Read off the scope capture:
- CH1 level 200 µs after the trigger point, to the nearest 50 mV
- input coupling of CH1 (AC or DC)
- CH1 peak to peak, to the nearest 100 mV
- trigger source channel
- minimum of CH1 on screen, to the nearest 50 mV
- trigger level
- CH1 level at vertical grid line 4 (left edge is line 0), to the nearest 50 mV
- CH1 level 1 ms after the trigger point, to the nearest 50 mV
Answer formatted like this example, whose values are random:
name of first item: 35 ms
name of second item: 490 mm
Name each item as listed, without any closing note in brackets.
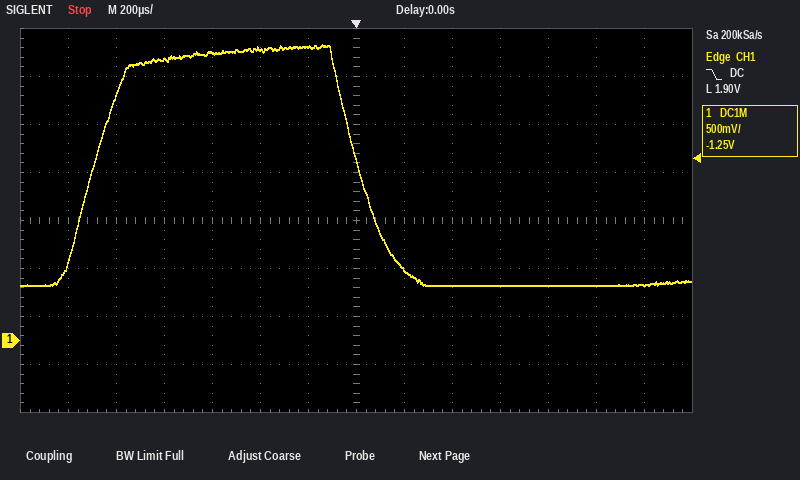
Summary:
CH1 level 200 µs after the trigger point, to the nearest 50 mV: 750 mV
input coupling of CH1: DC
CH1 peak to peak, to the nearest 100 mV: 2.50 V
trigger source channel: CH1
minimum of CH1 on screen, to the nearest 50 mV: 550 mV
trigger level: 1.90 V
CH1 level at vertical grid line 4 (left edge is line 0), to the nearest 50 mV: 3.00 V
CH1 level 1 ms after the trigger point, to the nearest 50 mV: 550 mV
